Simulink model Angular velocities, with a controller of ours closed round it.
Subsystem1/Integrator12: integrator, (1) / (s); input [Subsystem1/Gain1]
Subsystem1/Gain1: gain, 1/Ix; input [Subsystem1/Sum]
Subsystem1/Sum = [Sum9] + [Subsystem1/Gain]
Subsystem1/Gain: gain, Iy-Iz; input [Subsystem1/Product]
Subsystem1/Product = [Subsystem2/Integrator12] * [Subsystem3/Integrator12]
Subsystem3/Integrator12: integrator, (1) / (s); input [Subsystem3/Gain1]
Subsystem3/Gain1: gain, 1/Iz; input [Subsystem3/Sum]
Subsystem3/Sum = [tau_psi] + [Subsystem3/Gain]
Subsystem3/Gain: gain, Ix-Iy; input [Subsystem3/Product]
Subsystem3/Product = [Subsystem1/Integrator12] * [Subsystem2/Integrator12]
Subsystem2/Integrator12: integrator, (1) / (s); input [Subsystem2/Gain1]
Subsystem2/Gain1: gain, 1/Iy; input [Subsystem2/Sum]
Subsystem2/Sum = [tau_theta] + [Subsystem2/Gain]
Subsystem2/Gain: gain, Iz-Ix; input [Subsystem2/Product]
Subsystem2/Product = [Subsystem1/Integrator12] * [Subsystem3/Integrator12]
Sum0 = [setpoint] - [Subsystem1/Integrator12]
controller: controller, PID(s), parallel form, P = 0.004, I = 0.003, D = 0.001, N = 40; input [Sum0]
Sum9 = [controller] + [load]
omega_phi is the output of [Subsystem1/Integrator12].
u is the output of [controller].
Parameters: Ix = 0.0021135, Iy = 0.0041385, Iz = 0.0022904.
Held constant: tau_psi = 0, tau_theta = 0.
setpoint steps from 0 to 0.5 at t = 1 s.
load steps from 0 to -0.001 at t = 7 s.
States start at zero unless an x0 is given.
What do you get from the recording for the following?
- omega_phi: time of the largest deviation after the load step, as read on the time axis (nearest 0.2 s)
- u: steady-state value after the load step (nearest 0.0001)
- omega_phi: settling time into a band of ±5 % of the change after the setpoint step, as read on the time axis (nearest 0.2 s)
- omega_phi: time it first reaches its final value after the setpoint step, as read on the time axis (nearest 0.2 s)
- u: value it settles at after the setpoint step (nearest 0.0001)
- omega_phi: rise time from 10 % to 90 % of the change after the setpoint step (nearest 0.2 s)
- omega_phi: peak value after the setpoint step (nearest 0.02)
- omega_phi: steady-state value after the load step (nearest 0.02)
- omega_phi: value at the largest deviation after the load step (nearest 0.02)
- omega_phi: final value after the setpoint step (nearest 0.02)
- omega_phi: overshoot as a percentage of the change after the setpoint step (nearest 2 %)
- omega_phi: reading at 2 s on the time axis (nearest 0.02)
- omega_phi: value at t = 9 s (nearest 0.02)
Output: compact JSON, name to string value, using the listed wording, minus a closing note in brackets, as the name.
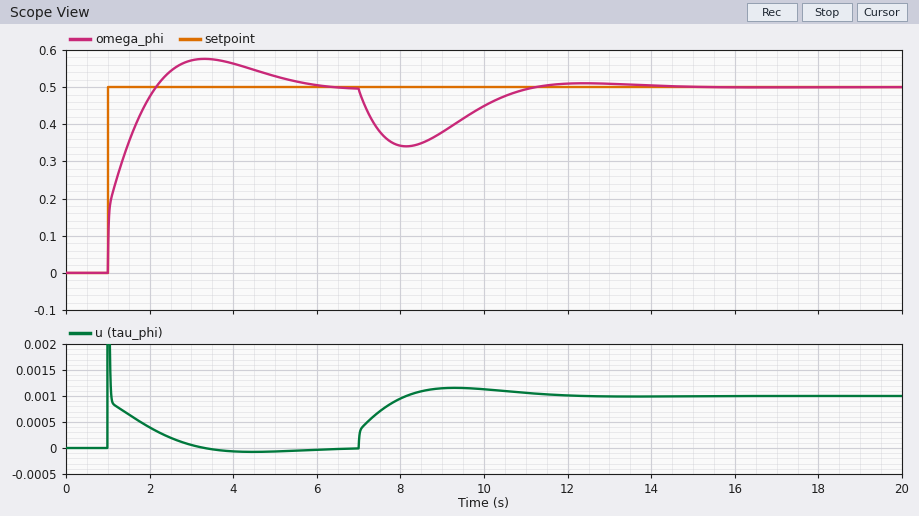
{"omega_phi: time of the largest deviation after the load step, as read on the time axis": "8.2 s", "u: steady-state value after the load step": "0.0010", "omega_phi: settling time into a band of ±5 % of the change after the setpoint step, as read on the time axis": "5.2 s", "omega_phi: time it first reaches its final value after the setpoint step, as read on the time axis": "2.2 s", "u: value it settles at after the setpoint step": "0.0000", "omega_phi: rise time from 10 % to 90 % of the change after the setpoint step": "0.8 s", "omega_phi: peak value after the setpoint step": "0.58", "omega_phi: steady-state value after the load step": "0.50", "omega_phi: value at the largest deviation after the load step": "0.34", "omega_phi: final value after the setpoint step": "0.50", "omega_phi: overshoot as a percentage of the change after the setpoint step": "16 %", "omega_phi: reading at 2 s on the time axis": "0.48", "omega_phi: value at t = 9 s": "0.38"}
